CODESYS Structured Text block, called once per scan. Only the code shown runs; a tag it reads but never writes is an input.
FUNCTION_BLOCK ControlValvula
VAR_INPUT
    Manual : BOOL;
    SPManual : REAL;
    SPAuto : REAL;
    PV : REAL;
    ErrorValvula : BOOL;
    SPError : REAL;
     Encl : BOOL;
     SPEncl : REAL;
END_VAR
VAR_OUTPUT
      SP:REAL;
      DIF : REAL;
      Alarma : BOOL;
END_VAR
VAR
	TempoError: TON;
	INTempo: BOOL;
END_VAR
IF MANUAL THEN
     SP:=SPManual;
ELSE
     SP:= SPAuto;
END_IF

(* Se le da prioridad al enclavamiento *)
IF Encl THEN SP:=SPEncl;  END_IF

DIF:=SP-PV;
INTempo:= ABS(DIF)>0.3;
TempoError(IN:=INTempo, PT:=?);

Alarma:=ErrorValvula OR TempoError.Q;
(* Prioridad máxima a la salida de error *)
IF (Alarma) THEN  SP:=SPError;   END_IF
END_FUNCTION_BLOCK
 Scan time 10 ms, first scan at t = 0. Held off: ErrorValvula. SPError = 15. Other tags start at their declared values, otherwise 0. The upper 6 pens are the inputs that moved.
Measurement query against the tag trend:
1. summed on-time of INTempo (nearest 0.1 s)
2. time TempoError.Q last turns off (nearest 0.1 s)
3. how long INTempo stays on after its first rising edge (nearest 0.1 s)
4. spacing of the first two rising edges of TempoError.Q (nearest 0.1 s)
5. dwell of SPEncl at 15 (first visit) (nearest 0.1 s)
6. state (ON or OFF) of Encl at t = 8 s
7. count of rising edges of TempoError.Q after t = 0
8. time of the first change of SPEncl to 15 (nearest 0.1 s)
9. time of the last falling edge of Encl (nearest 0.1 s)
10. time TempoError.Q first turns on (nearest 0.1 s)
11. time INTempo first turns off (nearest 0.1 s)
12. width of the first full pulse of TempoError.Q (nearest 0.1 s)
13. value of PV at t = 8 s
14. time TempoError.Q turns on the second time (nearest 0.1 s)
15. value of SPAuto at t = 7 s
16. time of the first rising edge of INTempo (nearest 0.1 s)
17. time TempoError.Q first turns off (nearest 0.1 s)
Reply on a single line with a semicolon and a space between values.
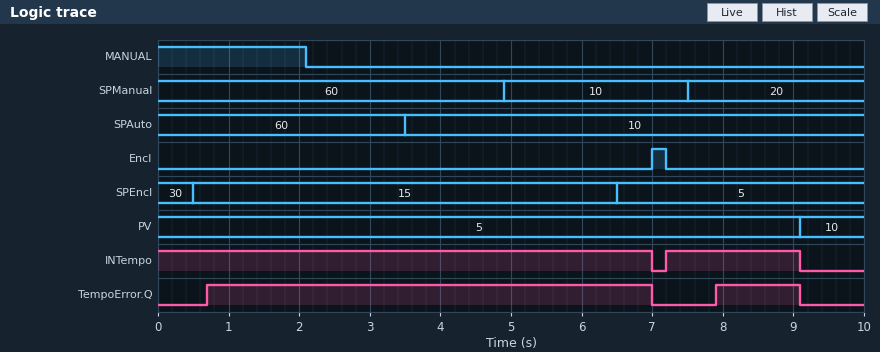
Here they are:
8.9 s; 9.1 s; 1.9 s; 7.2 s; 6.0 s; OFF; 2; 0.5 s; 7.2 s; 0.7 s; 7.0 s; 6.3 s; 5; 7.9 s; 10; 7.2 s; 7.0 s
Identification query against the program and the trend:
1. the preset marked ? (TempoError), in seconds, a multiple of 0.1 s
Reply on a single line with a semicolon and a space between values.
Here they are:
0.7 s
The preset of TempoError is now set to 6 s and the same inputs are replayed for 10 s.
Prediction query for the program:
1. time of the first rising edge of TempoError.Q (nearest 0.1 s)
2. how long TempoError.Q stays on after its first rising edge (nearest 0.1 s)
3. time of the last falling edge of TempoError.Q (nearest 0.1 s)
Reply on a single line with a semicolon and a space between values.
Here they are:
6.0 s; 1.0 s; 7.0 s
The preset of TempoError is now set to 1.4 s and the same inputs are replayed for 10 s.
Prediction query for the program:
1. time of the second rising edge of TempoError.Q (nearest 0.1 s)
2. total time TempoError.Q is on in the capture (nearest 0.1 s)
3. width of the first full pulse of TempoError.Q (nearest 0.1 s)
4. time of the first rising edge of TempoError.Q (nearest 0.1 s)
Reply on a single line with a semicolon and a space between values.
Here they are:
8.6 s; 6.1 s; 5.6 s; 1.4 s
